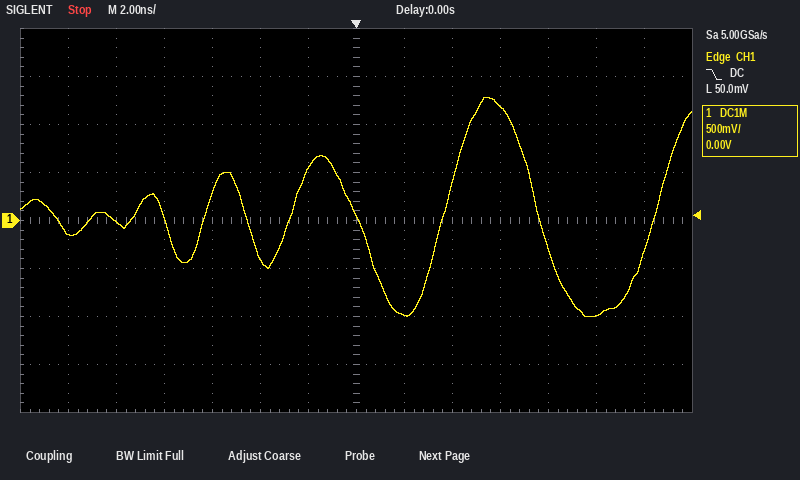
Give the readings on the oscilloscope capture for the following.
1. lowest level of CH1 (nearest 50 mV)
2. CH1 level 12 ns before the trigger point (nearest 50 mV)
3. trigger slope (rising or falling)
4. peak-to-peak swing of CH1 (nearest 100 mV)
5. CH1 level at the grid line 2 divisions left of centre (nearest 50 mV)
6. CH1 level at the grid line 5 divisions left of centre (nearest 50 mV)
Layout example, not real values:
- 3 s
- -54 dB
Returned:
- -1.00 V
- -150 mV
- falling
- 2.30 V
- -400 mV
- 0 mV
